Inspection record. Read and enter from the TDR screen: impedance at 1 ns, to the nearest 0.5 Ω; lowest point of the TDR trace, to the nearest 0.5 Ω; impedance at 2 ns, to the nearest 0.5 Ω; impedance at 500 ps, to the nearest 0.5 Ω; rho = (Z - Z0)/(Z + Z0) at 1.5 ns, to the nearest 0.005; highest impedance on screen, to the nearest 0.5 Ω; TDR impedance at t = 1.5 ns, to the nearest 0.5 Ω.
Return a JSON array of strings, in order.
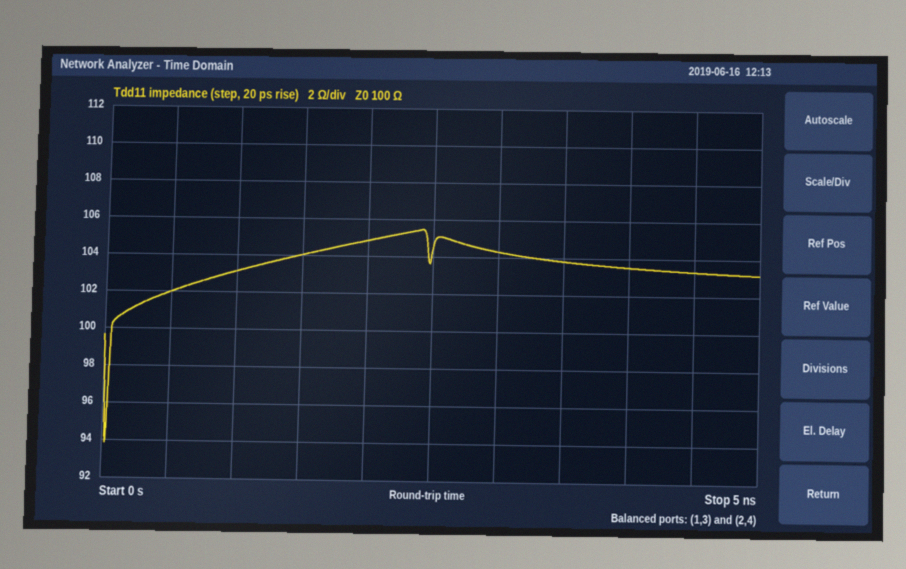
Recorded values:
["103.0 Ω", "94.0 Ω", "105.0 Ω", "102.0 Ω", "+0.020", "105.5 Ω", "104.0 Ω"]
